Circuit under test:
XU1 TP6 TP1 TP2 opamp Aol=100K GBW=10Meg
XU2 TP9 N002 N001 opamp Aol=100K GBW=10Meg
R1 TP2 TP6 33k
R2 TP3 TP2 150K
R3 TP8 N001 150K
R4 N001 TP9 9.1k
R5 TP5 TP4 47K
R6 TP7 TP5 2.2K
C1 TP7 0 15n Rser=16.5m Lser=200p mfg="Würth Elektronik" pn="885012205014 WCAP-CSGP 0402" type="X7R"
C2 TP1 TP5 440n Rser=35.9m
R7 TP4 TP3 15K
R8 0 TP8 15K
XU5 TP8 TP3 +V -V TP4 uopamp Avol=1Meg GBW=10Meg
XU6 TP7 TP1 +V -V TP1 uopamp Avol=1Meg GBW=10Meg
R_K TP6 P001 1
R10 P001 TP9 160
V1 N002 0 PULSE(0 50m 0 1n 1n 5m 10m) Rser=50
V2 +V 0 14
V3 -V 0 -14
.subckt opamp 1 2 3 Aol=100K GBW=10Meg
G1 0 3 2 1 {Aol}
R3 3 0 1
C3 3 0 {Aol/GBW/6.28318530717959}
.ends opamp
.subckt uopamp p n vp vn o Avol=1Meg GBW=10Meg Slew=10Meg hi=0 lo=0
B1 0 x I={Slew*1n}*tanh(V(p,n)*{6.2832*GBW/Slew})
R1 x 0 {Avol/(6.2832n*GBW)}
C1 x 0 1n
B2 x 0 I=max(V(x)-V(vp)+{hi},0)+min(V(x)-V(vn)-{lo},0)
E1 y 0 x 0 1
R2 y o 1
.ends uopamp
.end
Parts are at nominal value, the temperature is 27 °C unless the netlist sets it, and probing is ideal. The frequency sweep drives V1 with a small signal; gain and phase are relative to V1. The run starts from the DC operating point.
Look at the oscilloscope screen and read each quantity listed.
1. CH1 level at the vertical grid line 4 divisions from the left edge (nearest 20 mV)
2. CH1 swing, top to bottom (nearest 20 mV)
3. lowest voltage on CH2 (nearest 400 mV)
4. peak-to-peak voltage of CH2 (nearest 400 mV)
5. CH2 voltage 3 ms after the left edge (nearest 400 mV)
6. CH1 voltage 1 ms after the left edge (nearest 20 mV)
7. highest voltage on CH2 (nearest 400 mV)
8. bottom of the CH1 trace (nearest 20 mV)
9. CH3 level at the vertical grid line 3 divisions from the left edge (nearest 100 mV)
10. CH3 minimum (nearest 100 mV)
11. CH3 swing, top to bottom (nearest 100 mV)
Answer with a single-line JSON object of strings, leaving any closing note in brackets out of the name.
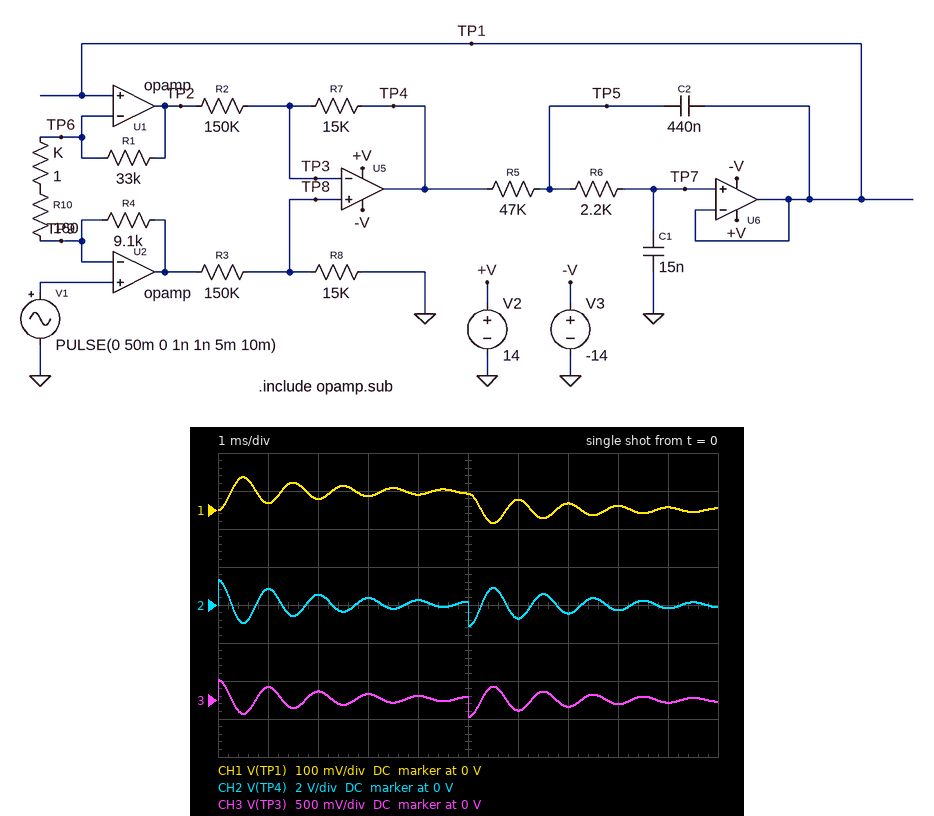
{"CH1 level at the vertical grid line 4 divisions from the left edge": "40 mV", "CH1 swing, top to bottom": "120 mV", "lowest voltage on CH2": "-1.2 V", "peak-to-peak voltage of CH2": "2.4 V", "CH2 voltage 3 ms after the left edge": "400 mV", "CH1 voltage 1 ms after the left edge": "20 mV", "highest voltage on CH2": "1.2 V", "bottom of the CH1 trace": "-40 mV", "CH3 level at the vertical grid line 3 divisions from the left edge": "100 mV", "CH3 minimum": "-200 mV", "CH3 swing, top to bottom": "500 mV"}
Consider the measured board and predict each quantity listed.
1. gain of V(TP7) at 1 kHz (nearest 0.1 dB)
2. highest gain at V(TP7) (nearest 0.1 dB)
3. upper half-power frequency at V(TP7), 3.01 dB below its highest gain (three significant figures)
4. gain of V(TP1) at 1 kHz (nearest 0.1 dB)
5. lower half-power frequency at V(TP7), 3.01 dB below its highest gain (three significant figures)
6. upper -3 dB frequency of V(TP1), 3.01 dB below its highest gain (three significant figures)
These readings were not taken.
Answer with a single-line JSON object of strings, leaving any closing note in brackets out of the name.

{"gain of V(TP7) at 1 kHz": "16.4 dB", "highest gain at V(TP7)": "16.4 dB", "upper half-power frequency at V(TP7), 3.01 dB below its highest gain": "1.07 kHz", "gain of V(TP1) at 1 kHz": "16.4 dB", "lower half-power frequency at V(TP7), 3.01 dB below its highest gain": "922 Hz", "upper -3 dB frequency of V(TP1), 3.01 dB below its highest gain": "1.07 kHz"}
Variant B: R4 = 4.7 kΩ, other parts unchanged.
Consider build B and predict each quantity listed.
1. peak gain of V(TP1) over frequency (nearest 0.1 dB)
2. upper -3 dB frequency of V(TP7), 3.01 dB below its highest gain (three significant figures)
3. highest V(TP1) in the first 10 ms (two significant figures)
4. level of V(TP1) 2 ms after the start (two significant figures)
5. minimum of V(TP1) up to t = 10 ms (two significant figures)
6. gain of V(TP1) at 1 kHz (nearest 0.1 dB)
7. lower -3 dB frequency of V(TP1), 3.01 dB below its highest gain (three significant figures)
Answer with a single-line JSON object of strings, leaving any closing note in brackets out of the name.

{"peak gain of V(TP1) over frequency": "15.6 dB", "upper -3 dB frequency of V(TP7), 3.01 dB below its highest gain": "1.02 kHz", "highest V(TP1) in the first 10 ms": "85 mV", "level of V(TP1) 2 ms after the start": "34 mV", "minimum of V(TP1) up to t = 10 ms": "-38 mV", "gain of V(TP1) at 1 kHz": "13.8 dB", "lower -3 dB frequency of V(TP1), 3.01 dB below its highest gain": "867 Hz"}
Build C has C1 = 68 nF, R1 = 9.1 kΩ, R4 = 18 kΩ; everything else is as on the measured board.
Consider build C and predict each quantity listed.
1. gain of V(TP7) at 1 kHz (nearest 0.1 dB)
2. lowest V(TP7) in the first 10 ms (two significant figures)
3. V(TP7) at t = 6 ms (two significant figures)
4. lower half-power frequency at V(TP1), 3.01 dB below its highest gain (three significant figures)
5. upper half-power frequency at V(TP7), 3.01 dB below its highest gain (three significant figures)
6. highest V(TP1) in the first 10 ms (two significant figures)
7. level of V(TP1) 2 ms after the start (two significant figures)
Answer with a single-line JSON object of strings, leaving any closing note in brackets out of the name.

{"gain of V(TP7) at 1 kHz": "-16.0 dB", "lowest V(TP7) in the first 10 ms": "-22 mV", "V(TP7) at t = 6 ms": "-15 mV", "lower half-power frequency at V(TP1), 3.01 dB below its highest gain": "262 Hz", "upper half-power frequency at V(TP7), 3.01 dB below its highest gain": "442 Hz", "highest V(TP1) in the first 10 ms": "70 mV", "level of V(TP1) 2 ms after the start": "51 mV"}
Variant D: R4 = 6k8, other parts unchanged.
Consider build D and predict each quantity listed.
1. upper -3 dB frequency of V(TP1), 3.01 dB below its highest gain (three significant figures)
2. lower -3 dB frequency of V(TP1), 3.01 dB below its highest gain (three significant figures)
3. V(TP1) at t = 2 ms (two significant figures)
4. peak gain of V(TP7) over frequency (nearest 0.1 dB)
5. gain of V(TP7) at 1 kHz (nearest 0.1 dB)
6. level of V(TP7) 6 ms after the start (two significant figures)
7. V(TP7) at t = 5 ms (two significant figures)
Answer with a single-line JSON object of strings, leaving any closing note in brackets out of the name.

{"upper -3 dB frequency of V(TP1), 3.01 dB below its highest gain": "1.04 kHz", "lower -3 dB frequency of V(TP1), 3.01 dB below its highest gain": "894 Hz", "V(TP1) at t = 2 ms": "31 mV", "peak gain of V(TP7) over frequency": "16.0 dB", "gain of V(TP7) at 1 kHz": "15.4 dB", "level of V(TP7) 6 ms after the start": "28 mV", "V(TP7) at t = 5 ms": "45 mV"}
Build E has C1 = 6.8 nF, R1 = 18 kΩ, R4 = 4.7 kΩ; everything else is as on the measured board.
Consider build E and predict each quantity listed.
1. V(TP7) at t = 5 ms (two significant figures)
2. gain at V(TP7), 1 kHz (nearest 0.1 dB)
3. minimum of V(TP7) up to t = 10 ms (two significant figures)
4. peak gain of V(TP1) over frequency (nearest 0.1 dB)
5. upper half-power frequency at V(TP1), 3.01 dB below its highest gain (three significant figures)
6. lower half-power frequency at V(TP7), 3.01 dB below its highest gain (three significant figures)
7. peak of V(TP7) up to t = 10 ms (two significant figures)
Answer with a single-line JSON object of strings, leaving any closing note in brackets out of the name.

{"V(TP7) at t = 5 ms": "51 mV", "gain at V(TP7), 1 kHz": "12.1 dB", "minimum of V(TP7) up to t = 10 ms": "-41 mV", "peak gain of V(TP1) over frequency": "16.5 dB", "upper half-power frequency at V(TP1), 3.01 dB below its highest gain": "1.18 kHz", "lower half-power frequency at V(TP7), 3.01 dB below its highest gain": "1.03 kHz", "peak of V(TP7) up to t = 10 ms": "84 mV"}
